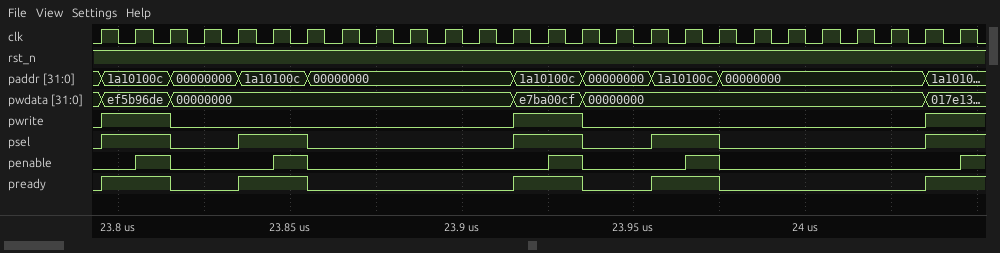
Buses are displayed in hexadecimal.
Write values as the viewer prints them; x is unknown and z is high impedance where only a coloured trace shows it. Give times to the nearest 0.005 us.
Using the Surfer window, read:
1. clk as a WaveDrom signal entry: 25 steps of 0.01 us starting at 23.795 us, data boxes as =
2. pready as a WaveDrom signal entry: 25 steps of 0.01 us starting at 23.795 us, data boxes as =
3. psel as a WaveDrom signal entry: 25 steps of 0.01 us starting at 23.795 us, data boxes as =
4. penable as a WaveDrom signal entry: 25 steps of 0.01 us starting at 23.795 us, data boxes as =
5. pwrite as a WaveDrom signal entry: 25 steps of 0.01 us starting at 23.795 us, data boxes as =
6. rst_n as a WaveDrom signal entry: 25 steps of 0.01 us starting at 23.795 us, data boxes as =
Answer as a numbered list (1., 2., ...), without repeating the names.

1. {name: 'clk', wave: 'p........................'}
2. {name: 'pready', wave: '1.0.1.0.....1.0.1.0.....1'}
3. {name: 'psel', wave: '1.0.1.0.....1.0.1.0.....1'}
4. {name: 'penable', wave: '010..10......10..10......'}
5. {name: 'pwrite', wave: '1.0.........1.0.........1'}
6. {name: 'rst_n', wave: '1........................'}
